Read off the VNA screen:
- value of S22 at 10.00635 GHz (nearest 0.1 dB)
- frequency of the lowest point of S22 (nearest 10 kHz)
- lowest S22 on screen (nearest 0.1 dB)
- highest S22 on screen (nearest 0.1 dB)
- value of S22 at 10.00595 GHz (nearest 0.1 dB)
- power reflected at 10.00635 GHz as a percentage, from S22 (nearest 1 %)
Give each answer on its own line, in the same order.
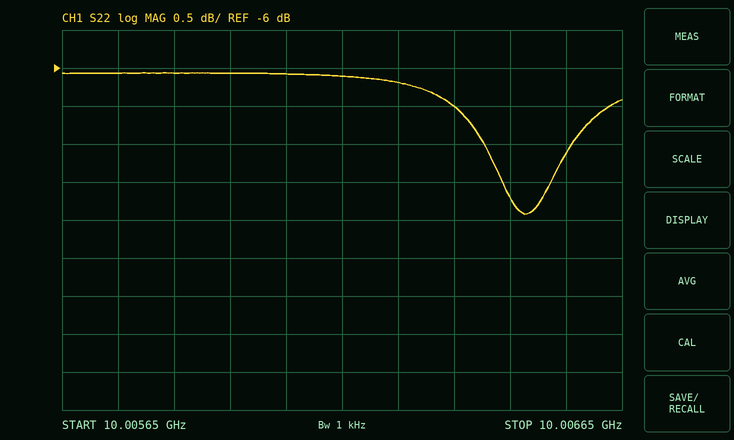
-6.5 dB
10.00648 GHz
-7.9 dB
-6.1 dB
-6.1 dB
22 %
